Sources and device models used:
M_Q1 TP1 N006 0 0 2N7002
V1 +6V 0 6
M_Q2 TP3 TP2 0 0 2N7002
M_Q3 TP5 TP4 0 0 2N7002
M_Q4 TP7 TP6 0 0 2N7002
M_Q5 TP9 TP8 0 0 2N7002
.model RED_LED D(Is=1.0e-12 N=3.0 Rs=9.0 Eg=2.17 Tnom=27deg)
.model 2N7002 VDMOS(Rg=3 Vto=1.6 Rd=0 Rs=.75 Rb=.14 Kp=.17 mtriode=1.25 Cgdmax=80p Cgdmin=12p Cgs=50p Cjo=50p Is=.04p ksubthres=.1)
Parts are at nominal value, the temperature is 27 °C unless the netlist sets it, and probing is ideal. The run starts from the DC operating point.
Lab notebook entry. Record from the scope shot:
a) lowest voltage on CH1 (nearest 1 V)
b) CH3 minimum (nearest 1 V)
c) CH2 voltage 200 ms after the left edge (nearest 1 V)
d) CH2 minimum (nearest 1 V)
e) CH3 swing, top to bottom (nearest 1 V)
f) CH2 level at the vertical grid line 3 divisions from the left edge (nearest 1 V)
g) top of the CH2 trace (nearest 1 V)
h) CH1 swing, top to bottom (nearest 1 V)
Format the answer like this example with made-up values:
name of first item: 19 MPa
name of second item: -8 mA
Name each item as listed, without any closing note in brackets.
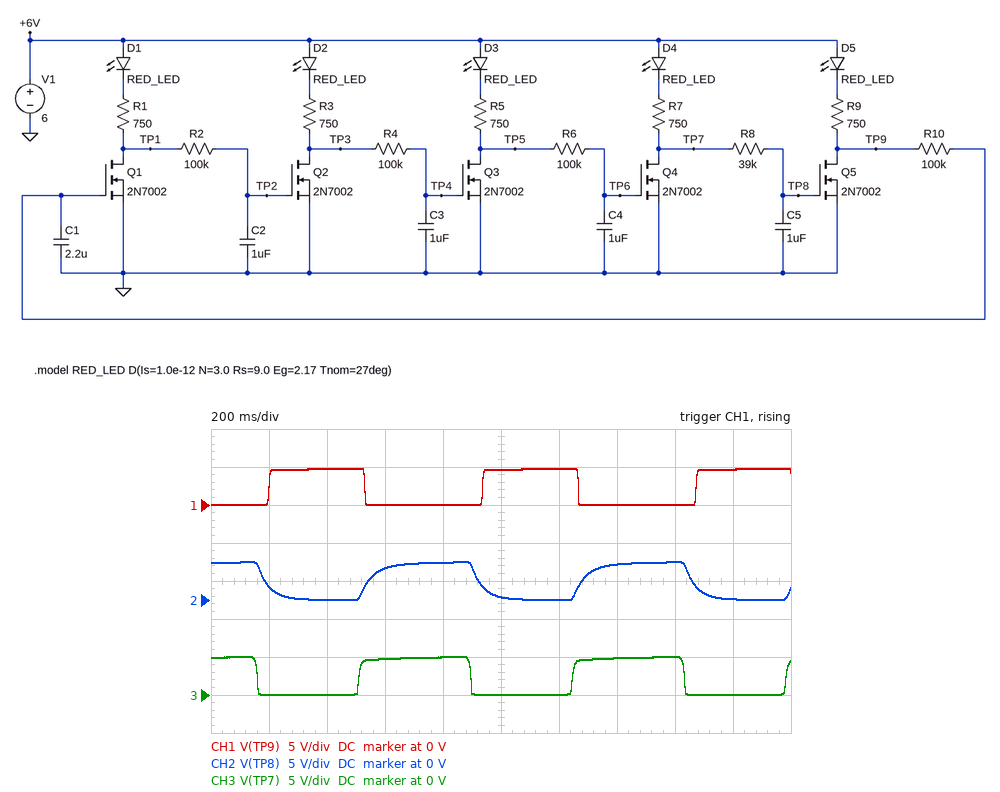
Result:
lowest voltage on CH1: 0 V
CH3 minimum: 0 V
CH2 voltage 200 ms after the left edge: 2 V
CH2 minimum: 0 V
CH3 swing, top to bottom: 5 V
CH2 level at the vertical grid line 3 divisions from the left edge: 4 V
top of the CH2 trace: 5 V
CH1 swing, top to bottom: 5 V
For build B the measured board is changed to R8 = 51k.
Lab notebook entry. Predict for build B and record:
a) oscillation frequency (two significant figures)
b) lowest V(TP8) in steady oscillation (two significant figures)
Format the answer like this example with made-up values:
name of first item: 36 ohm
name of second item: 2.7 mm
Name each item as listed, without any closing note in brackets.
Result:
oscillation frequency: 1.3 Hz
lowest V(TP8) in steady oscillation: 26 mV
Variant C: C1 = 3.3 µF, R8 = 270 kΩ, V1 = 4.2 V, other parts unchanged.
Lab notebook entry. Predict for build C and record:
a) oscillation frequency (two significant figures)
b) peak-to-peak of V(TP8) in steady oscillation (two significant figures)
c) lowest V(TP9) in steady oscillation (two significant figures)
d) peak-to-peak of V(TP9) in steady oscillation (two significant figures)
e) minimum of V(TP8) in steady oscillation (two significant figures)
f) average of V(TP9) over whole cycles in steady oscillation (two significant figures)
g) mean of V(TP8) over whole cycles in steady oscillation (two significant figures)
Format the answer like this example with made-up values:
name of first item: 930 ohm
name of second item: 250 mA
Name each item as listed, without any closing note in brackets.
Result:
oscillation frequency: 890 mHz
peak-to-peak of V(TP8) in steady oscillation: 2.3 V
lowest V(TP9) in steady oscillation: 17 mV
peak-to-peak of V(TP9) in steady oscillation: 3.0 V
minimum of V(TP8) in steady oscillation: 370 mV
average of V(TP9) over whole cycles in steady oscillation: 1.6 V
mean of V(TP8) over whole cycles in steady oscillation: 1.5 V
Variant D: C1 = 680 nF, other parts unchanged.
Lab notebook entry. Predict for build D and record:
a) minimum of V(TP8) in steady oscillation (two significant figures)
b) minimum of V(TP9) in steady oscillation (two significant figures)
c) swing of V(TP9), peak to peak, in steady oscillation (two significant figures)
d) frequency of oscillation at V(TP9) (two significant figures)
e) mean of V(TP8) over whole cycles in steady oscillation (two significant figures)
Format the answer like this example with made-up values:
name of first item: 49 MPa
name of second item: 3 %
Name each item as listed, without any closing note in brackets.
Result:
minimum of V(TP8) in steady oscillation: 26 mV
minimum of V(TP9) in steady oscillation: 12 mV
swing of V(TP9), peak to peak, in steady oscillation: 4.9 V
frequency of oscillation at V(TP9): 1.8 Hz
mean of V(TP8) over whole cycles in steady oscillation: 2.3 V
